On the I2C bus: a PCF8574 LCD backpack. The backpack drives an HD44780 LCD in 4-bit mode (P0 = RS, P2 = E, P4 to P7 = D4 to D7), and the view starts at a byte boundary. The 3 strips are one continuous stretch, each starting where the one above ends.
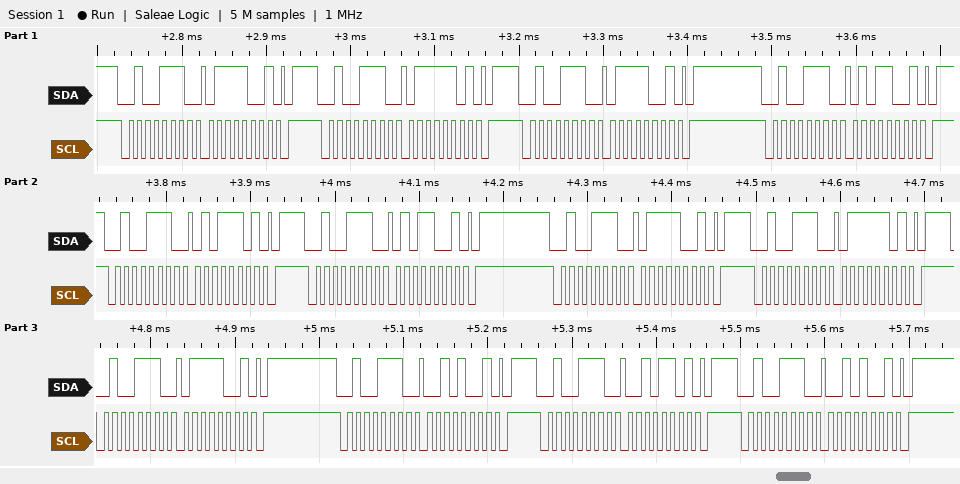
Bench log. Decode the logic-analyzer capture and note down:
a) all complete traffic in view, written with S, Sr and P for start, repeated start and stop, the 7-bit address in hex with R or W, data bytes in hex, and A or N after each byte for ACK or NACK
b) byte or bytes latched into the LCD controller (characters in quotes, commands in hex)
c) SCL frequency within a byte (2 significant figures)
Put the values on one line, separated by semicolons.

S 27W A 79 A P S 27W A 7D A P S 27W A 79 A P S 27W A 59 A P S 27W A 5D A P S 27W A 59 A P S 27W A 79 A P S 27W A 7D A P S 27W A 79 A P S 27W A 29 A P S 27W A 2D A P S 27W A 29 A P; 'u' 'r'; 100 kHz
